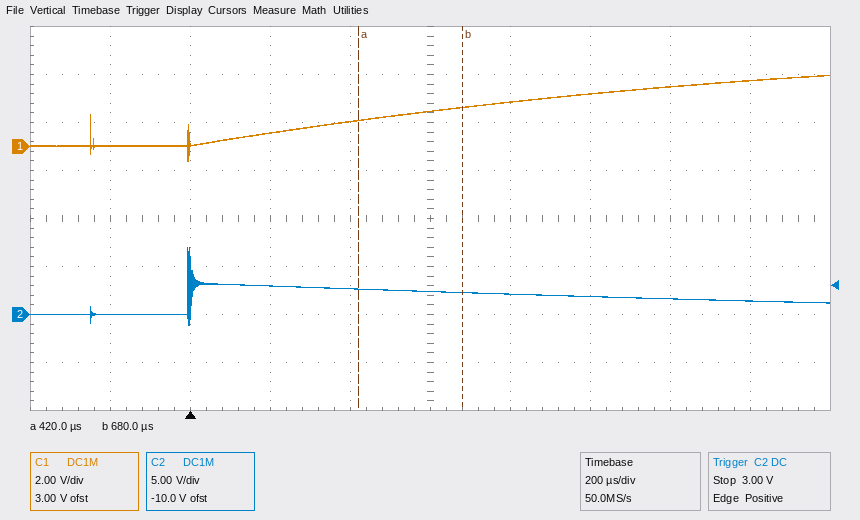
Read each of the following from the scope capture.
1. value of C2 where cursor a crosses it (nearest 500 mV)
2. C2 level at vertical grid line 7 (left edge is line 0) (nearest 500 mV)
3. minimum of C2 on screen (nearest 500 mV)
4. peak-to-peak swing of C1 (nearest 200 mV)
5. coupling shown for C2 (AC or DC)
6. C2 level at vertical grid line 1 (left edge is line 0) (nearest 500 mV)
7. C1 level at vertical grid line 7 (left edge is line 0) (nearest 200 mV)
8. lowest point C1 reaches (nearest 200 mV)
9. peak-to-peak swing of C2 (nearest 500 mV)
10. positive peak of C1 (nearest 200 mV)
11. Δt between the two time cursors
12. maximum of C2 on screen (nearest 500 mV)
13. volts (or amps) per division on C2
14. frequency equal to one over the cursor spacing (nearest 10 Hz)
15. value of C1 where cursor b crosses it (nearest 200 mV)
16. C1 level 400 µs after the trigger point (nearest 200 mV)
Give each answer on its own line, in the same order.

2.5 V
2.0 V
-1.0 V
3.6 V
DC
0.0 V
2.2 V
-600 mV
8.0 V
3.0 V
260 µs
7.0 V
5 V
3.85 kHz
1.6 V
1.0 V
